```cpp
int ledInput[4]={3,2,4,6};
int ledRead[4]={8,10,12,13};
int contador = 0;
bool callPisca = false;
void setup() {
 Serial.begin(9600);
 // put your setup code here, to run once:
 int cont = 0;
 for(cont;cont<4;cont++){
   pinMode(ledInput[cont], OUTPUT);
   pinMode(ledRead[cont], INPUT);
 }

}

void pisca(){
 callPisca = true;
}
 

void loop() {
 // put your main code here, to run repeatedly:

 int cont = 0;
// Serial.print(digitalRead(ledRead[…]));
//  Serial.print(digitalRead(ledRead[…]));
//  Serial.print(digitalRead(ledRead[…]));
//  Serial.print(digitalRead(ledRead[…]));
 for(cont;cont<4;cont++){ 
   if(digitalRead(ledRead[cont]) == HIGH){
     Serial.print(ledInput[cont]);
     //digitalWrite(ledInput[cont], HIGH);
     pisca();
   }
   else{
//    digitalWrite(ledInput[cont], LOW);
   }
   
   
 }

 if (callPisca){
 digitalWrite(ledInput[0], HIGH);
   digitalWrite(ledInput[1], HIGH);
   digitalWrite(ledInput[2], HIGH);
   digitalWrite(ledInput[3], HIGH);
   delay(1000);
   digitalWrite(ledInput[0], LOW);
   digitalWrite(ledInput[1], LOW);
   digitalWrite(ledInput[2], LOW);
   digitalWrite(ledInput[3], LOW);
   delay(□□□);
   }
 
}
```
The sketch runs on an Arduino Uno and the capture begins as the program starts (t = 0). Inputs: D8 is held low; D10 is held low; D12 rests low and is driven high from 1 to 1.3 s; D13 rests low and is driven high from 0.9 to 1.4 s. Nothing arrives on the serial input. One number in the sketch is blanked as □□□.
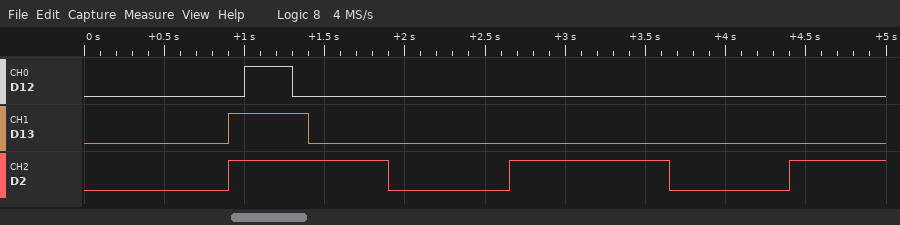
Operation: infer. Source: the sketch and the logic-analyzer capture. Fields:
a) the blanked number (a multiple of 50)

750
